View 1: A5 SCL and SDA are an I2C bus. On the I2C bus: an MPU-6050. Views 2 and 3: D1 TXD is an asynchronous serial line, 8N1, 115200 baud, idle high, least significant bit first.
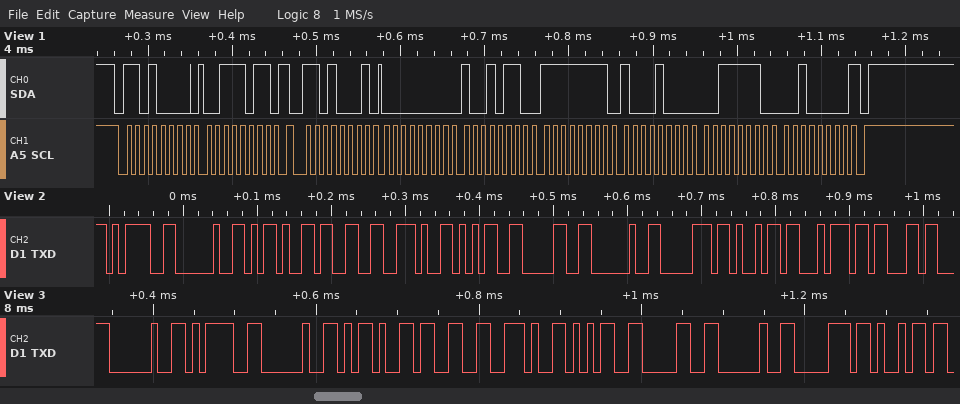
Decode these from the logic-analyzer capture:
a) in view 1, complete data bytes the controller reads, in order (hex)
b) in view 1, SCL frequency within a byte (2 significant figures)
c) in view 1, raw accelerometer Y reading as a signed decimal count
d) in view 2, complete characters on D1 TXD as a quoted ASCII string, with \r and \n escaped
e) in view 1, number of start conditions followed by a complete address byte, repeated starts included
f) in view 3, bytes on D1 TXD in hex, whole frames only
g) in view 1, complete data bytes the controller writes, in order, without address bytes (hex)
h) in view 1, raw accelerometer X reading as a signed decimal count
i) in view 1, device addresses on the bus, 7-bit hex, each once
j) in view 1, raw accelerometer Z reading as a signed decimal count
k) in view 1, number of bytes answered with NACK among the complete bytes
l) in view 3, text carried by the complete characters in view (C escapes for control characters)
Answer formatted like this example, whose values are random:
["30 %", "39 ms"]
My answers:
["00 96 FF 88 3E 20", "100 kHz", "-120", "\"= -3.50 pitc\"", "2", "0x20 0x3D 0x20 0x2D 0x33 0x2E 0x35 0x30 0x20 0x70 0x69", "3B", "150", "0x68", "15904", "1", "\" = -3.50 pi\""]
